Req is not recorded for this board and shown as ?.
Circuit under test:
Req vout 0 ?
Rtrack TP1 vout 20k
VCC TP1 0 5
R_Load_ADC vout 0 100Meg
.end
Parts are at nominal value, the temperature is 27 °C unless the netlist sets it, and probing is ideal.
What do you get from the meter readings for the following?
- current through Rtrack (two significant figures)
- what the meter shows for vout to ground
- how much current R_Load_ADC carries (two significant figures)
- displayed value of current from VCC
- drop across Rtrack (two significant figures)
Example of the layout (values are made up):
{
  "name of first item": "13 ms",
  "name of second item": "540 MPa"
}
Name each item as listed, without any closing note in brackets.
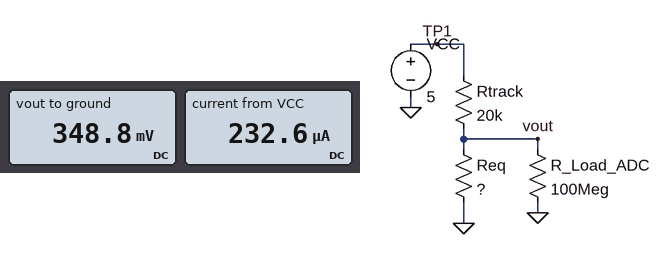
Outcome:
{
  "current through Rtrack": "230 µA",
  "what the meter shows for vout to ground": "348.8 mV",
  "how much current R_Load_ADC carries": "3.5 nA",
  "displayed value of current from VCC": "232.6 µA",
  "drop across Rtrack": "4.7 V"
}
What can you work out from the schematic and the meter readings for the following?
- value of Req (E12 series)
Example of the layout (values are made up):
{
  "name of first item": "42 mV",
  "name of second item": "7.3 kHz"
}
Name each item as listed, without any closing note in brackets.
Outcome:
{
  "value of Req": "1.5 kΩ"
}
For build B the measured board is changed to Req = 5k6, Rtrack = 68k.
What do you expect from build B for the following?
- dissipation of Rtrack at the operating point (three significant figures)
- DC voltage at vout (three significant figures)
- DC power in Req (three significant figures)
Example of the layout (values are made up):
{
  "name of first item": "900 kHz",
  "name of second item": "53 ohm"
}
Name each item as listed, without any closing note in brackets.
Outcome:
{
  "dissipation of Rtrack at the operating point": "314 µW",
  "DC voltage at vout": "380 mV",
  "DC power in Req": "25.8 µW"
}
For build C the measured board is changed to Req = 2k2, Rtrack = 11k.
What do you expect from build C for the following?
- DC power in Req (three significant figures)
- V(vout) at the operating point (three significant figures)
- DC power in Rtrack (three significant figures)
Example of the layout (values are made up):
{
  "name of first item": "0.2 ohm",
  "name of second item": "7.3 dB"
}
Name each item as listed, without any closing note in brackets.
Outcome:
{
  "DC power in Req": "316 µW",
  "V(vout) at the operating point": "833 mV",
  "DC power in Rtrack": "1.58 mW"
}
